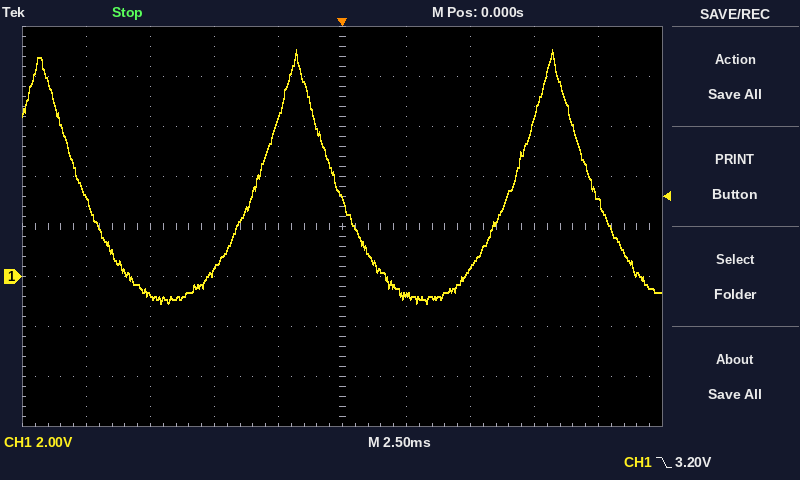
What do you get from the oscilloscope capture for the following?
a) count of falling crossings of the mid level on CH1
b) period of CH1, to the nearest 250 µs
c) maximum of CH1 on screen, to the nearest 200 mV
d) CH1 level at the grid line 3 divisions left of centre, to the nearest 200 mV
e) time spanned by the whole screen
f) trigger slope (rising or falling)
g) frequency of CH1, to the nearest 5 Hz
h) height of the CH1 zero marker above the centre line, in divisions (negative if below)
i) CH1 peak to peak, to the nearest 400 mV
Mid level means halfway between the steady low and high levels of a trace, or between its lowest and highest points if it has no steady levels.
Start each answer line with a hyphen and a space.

- 3
- 10.00 ms
- 9.0 V
- -800 mV
- 25 ms
- falling
- 100 Hz
- -1.0 div
- 10.0 V
